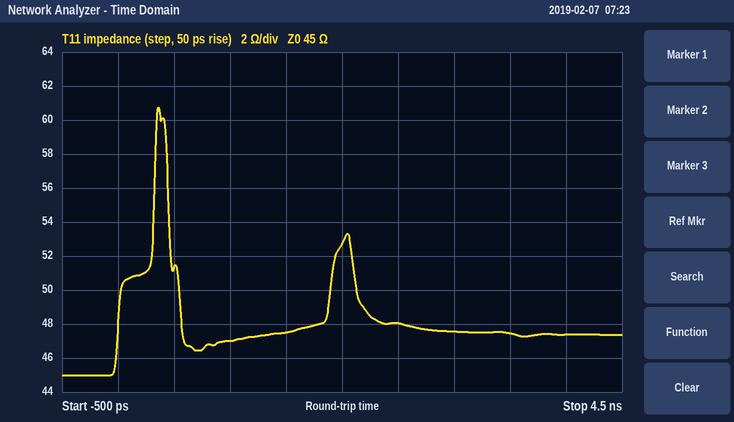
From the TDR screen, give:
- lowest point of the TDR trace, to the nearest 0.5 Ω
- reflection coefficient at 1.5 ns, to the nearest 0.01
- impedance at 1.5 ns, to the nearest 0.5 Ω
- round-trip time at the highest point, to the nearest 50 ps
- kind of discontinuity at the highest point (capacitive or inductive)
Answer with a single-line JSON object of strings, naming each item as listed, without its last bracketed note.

{"lowest point of the TDR trace, to the nearest 0.5 Ω": "45.0 Ω", "reflection coefficient at 1.5 ns, to the nearest 0.01": "+0.03", "impedance at 1.5 ns, to the nearest 0.5 Ω": "47.5 Ω", "round-trip time at the highest point, to the nearest 50 ps": "350 ps", "kind of discontinuity at the highest point": "inductive"}
